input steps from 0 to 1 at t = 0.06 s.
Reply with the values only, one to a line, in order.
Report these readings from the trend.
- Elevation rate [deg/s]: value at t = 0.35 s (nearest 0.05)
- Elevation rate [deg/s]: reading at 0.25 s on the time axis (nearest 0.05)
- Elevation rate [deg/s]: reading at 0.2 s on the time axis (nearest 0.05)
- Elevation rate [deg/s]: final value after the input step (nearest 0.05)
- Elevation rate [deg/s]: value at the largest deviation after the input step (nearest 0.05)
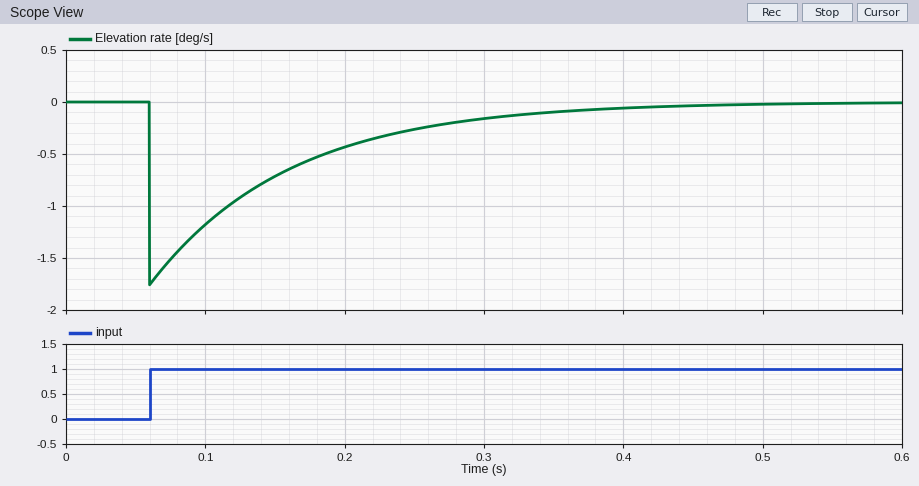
-0.10
-0.25
-0.45
0.00
-1.75
